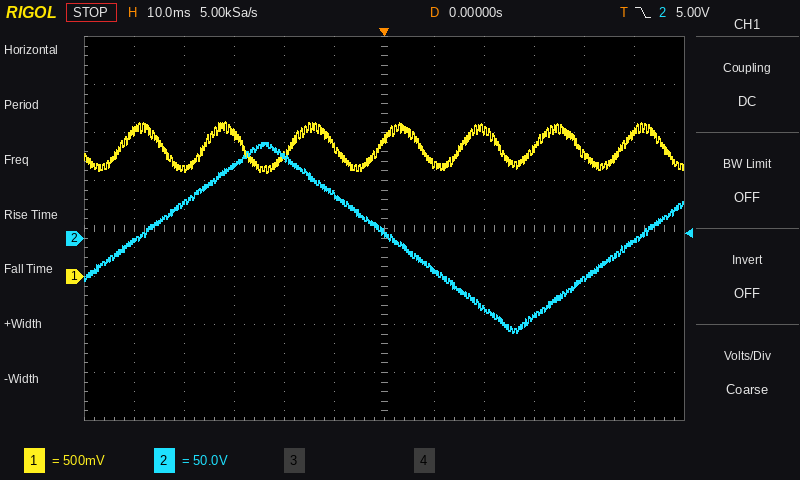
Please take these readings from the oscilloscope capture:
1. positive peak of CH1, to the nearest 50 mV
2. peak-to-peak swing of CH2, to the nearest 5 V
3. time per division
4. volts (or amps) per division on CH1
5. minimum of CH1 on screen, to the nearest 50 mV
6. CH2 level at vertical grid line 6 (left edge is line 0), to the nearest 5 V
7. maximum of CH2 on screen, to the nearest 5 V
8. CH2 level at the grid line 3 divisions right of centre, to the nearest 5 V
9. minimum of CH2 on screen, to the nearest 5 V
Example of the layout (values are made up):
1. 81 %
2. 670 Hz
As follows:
1. 1.60 V
2. 200 V
3. 10 ms
4. 500 mV
5. 1.10 V
6. 5 V
7. 100 V
8. -80 V
9. -100 V
